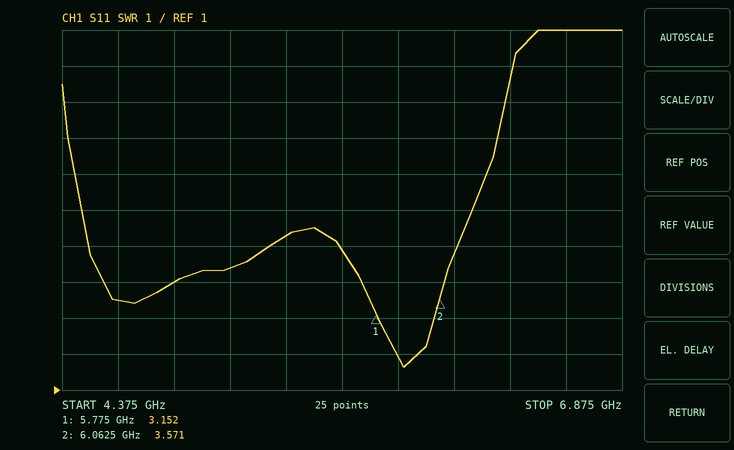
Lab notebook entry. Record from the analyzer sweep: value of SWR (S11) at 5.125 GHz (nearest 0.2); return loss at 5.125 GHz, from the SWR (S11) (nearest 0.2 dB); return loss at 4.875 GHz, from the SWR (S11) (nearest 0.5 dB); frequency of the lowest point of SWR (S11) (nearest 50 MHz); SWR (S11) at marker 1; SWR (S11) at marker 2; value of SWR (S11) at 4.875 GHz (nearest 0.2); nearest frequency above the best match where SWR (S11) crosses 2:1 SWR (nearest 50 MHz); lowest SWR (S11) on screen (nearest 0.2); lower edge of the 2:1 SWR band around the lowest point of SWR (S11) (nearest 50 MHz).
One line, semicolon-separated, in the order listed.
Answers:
4.4; 4.0 dB; 4.5 dB; 5.90 GHz; 3.152; 3.571; 4.0; 5.95 GHz; 1.6; 5.85 GHz
